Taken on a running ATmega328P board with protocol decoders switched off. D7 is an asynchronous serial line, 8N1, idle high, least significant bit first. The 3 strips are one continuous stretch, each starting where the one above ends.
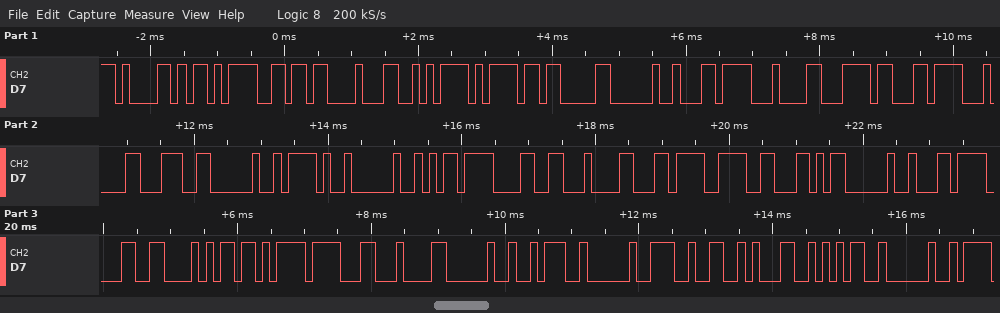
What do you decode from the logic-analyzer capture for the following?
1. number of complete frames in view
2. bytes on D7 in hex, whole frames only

37
61 EB B6 88 EA BD 83 20 EC 84 BC EC 84 9C 20 2F 20 ED 98 84 EC 9E AC 20 EC 98 A8 EB 8F 84 20 3A 20 32 31 35 20
